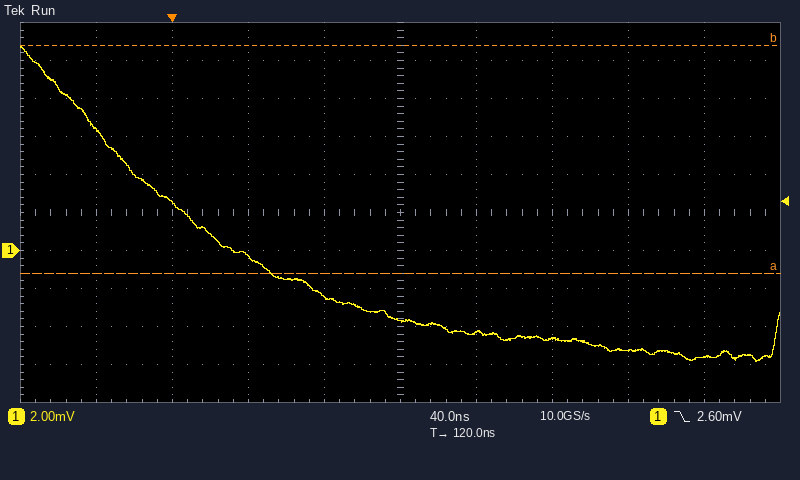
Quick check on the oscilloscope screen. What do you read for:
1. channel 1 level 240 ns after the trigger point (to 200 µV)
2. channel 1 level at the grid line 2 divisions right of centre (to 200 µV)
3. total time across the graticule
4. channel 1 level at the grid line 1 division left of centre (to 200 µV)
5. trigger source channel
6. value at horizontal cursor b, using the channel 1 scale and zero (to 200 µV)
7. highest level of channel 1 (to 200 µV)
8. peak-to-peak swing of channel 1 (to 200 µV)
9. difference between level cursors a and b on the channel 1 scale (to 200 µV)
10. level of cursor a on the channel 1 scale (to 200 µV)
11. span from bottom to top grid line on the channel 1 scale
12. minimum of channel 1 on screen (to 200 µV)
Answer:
-5.2 mV
-4.6 mV
400 ns
-2.4 mV
channel 1
10.8 mV
10.8 mV
16.6 mV
12.0 mV
-1.2 mV
20 mV
-5.8 mV
